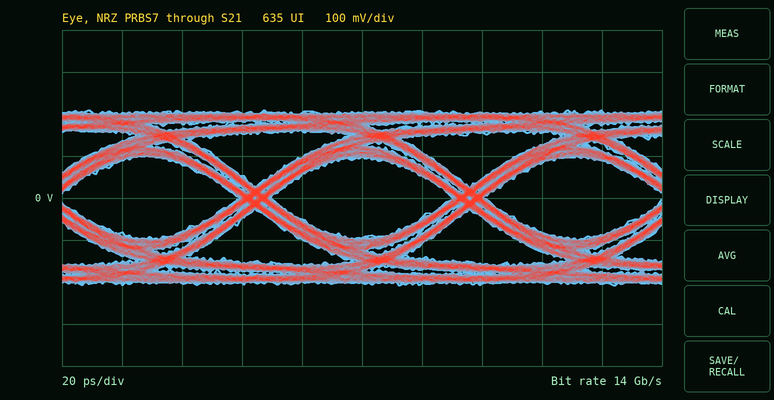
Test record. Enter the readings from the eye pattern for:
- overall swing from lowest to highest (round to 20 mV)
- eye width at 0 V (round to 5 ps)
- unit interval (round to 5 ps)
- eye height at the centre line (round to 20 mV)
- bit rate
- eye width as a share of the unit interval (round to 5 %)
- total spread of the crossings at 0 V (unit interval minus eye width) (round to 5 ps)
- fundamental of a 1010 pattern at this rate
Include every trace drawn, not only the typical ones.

420 mV
60 ps
70 ps
200 mV
14 Gb/s
85 %
10 ps
7 GHz
